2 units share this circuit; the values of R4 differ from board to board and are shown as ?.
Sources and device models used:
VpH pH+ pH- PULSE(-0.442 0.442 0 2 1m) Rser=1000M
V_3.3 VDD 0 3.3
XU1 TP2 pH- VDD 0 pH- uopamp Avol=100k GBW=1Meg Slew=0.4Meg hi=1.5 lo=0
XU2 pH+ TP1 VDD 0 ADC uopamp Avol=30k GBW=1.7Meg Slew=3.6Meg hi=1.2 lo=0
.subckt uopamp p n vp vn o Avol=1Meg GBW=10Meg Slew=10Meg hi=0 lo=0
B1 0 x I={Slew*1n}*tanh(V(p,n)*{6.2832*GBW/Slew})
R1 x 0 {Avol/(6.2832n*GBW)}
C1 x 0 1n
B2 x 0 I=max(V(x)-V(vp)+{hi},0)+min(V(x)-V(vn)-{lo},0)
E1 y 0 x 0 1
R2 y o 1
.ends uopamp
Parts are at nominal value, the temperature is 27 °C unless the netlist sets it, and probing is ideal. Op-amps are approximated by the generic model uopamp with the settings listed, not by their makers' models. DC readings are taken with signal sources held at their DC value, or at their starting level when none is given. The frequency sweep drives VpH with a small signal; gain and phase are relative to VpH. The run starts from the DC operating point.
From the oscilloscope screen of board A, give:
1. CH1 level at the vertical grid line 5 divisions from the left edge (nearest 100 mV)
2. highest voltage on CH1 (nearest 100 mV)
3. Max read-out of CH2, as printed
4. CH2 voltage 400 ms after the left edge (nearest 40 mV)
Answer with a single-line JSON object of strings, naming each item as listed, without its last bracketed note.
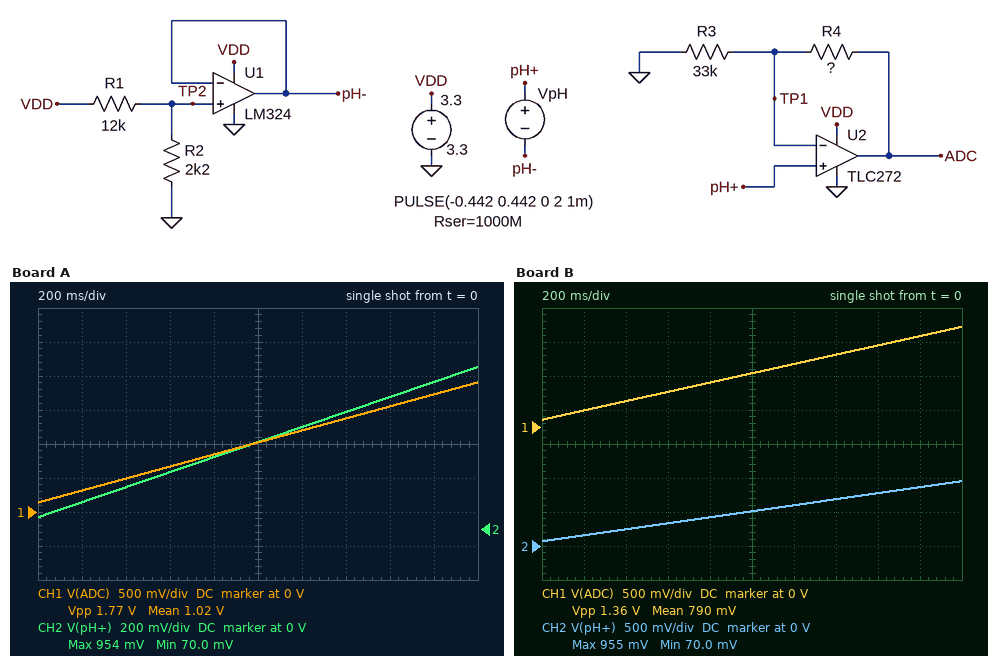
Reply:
{"CH1 level at the vertical grid line 5 divisions from the left edge": "1.0 V", "highest voltage on CH1": "1.9 V", "Max read-out of CH2, as printed": "954 mV", "CH2 voltage 400 ms after the left edge": "240 mV"}
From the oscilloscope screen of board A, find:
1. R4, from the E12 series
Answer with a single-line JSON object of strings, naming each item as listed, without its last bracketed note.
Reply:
{"R4, from the E12 series": "33 kΩ"}
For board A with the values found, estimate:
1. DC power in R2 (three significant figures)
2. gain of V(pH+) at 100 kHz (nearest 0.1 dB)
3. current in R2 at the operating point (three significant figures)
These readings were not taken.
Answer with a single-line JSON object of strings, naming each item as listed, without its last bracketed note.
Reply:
{"DC power in R2": "119 µW", "gain of V(pH+) at 100 kHz": "0 dB", "current in R2 at the operating point": "232 µA"}
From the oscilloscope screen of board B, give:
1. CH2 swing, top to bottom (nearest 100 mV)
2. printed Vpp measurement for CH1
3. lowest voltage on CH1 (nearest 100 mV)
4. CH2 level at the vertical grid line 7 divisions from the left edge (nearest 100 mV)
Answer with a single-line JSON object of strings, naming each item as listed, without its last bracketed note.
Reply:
{"CH2 swing, top to bottom": "900 mV", "printed Vpp measurement for CH1": "1.36 V", "lowest voltage on CH1": "100 mV", "CH2 level at the vertical grid line 7 divisions from the left edge": "700 mV"}
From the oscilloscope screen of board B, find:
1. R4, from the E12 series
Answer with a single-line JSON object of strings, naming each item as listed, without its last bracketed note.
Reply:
{"R4, from the E12 series": "18 kΩ"}
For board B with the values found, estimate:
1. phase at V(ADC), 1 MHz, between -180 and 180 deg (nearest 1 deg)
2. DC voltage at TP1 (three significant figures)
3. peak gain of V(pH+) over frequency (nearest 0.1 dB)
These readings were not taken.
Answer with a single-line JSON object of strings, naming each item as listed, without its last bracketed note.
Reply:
{"phase at V(ADC), 1 MHz, between -180 and 180 deg": "-42 deg", "DC voltage at TP1": "69.3 mV", "peak gain of V(pH+) over frequency": "0 dB"}
